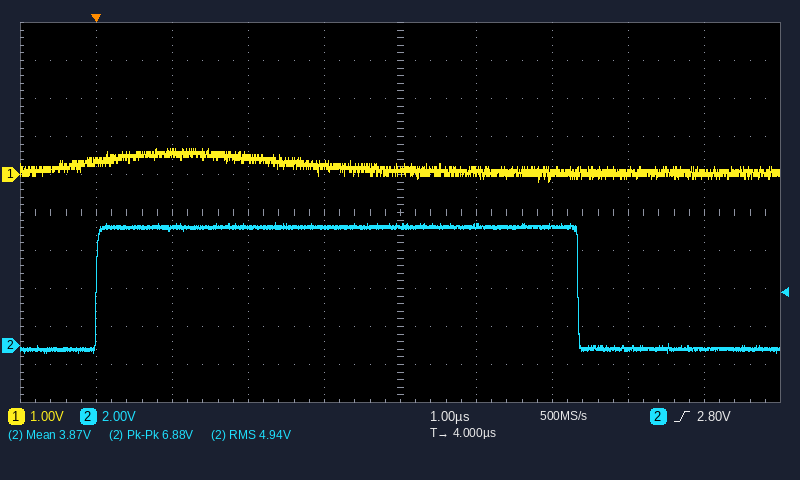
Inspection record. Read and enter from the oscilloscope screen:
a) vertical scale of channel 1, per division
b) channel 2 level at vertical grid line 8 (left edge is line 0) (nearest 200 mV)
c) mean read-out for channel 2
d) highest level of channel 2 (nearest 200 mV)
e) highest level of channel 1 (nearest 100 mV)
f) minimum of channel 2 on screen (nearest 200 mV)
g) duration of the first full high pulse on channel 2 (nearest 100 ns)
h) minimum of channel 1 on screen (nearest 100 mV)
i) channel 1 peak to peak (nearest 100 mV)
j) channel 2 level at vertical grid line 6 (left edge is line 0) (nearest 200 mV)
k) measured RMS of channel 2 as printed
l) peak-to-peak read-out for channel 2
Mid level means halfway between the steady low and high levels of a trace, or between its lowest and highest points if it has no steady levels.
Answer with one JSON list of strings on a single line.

["1 V", "-200 mV", "3.87 V", "6.4 V", "700 mV", "-400 mV", "6.3 µs", "-200 mV", "900 mV", "6.2 V", "4.94 V", "6.88 V"]
